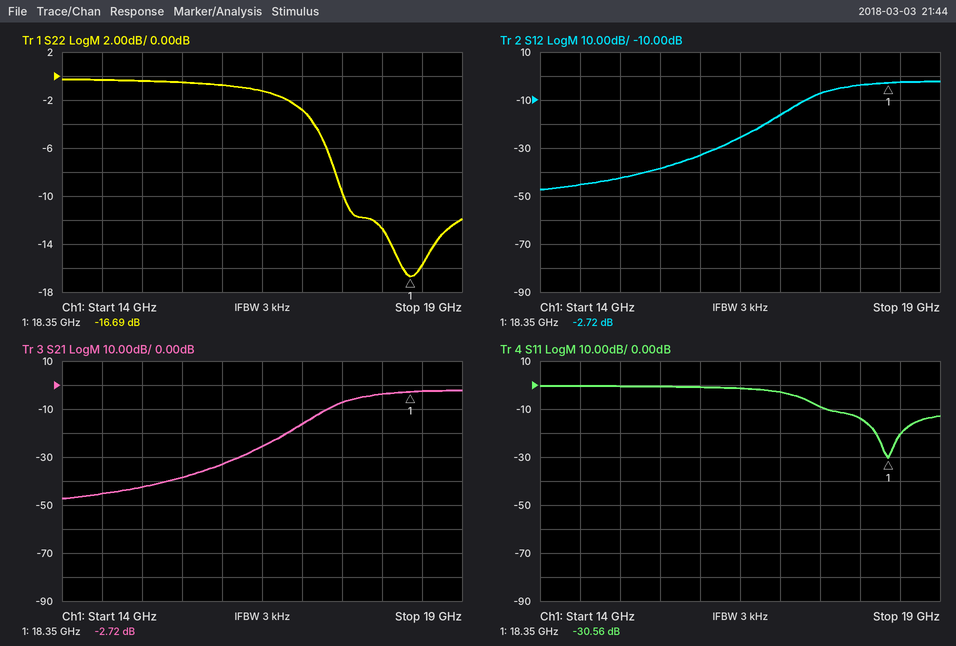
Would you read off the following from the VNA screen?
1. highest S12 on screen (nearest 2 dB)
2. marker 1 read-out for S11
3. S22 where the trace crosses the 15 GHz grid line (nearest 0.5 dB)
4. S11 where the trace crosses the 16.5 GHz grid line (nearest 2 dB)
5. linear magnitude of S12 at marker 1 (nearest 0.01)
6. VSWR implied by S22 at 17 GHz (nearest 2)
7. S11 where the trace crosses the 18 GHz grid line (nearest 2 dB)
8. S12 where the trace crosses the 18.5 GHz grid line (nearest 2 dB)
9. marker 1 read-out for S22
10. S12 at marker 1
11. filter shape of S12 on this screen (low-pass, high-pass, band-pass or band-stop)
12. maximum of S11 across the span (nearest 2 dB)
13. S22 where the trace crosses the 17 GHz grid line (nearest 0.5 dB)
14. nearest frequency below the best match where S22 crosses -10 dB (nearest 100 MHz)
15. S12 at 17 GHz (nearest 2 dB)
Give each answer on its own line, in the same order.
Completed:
-2 dB
-30.56 dB
-0.5 dB
-2 dB
0.73
6
-14 dB
-2 dB
-16.69 dB
-2.72 dB
high-pass
0 dB
-3.0 dB
17.5 GHz
-16 dB
